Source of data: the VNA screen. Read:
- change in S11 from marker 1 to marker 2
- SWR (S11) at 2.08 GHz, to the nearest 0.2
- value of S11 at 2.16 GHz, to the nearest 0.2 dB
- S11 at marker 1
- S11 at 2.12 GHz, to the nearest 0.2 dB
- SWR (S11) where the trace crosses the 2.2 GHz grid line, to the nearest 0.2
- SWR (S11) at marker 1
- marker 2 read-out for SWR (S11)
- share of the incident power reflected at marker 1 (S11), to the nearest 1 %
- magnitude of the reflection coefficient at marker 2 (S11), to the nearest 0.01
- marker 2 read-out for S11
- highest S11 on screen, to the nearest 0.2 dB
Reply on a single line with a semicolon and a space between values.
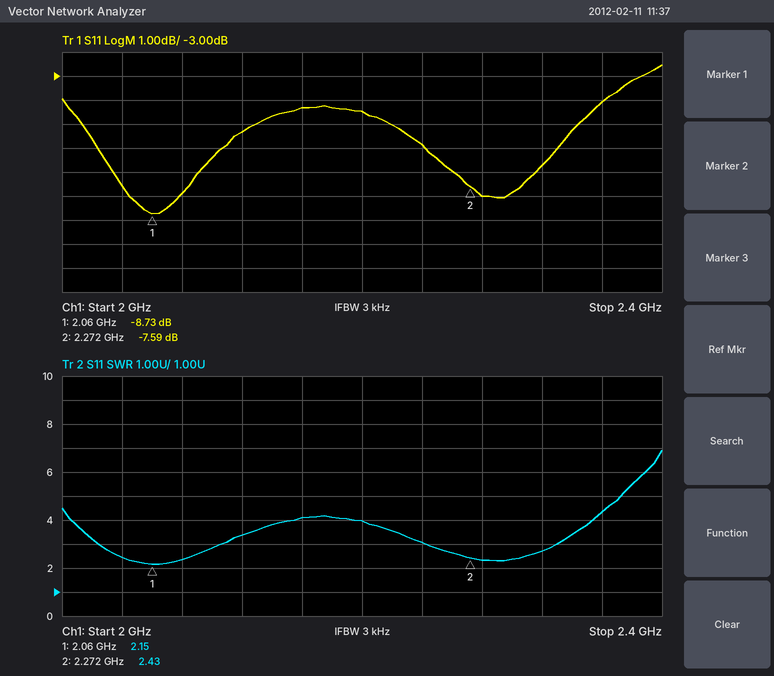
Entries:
1.14 dB; 2.4; -4.4 dB; -8.73 dB; -5.4 dB; 4.0; 2.15; 2.43; 13 %; 0.42; -7.59 dB; -2.6 dB
